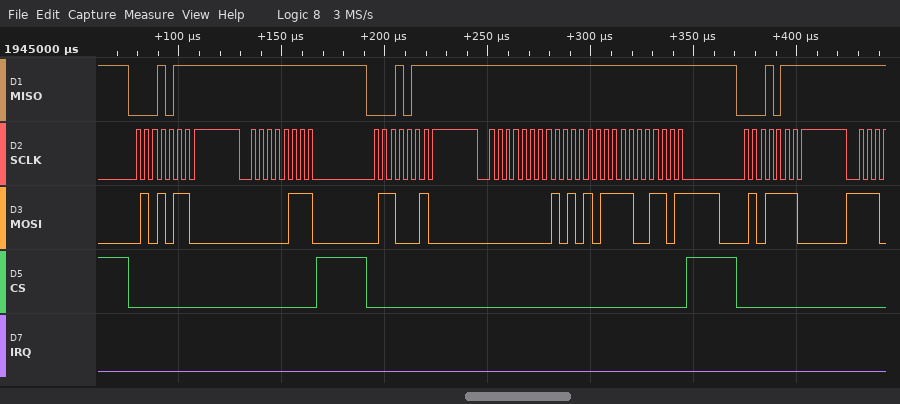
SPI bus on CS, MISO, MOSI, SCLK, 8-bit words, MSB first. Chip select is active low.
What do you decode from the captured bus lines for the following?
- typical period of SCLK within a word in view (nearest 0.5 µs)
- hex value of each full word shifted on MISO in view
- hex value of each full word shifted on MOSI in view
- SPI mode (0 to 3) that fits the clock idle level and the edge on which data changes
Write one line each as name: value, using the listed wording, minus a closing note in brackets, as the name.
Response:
typical period of SCLK within a word in view: 4 µs
hex value of each full word shifted on MISO in view: 17, FF, 17, FF, FF, FF, 17
hex value of each full word shifted on MOSI in view: 56, 07, 62, 00, AB, CD, 5E
SPI mode (0 to 3) that fits the clock idle level and the edge on which data changes: 0
